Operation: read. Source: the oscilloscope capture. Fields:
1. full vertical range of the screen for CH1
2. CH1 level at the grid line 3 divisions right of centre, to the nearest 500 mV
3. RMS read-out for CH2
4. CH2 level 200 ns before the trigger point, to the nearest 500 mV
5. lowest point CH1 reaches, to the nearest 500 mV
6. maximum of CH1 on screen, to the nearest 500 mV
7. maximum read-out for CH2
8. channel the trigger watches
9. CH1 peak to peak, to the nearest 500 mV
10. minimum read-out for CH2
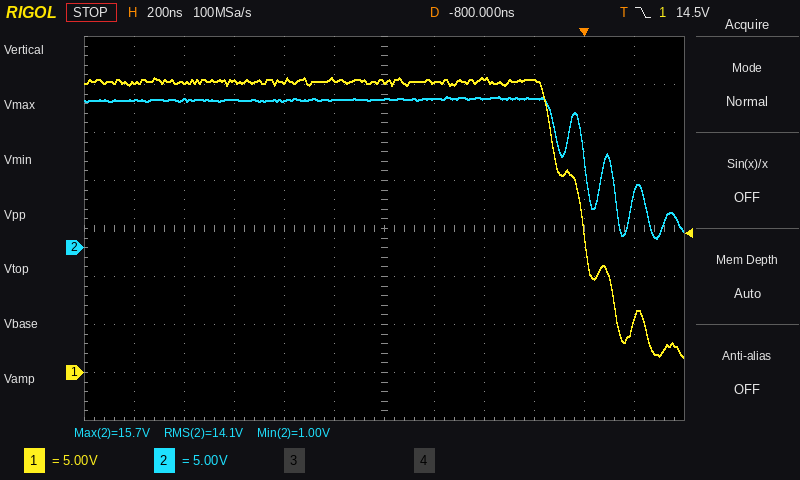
40 V
30.5 V
14.1 V
15.5 V
1.5 V
30.5 V
15.7 V
CH1
29.0 V
1.00 V
